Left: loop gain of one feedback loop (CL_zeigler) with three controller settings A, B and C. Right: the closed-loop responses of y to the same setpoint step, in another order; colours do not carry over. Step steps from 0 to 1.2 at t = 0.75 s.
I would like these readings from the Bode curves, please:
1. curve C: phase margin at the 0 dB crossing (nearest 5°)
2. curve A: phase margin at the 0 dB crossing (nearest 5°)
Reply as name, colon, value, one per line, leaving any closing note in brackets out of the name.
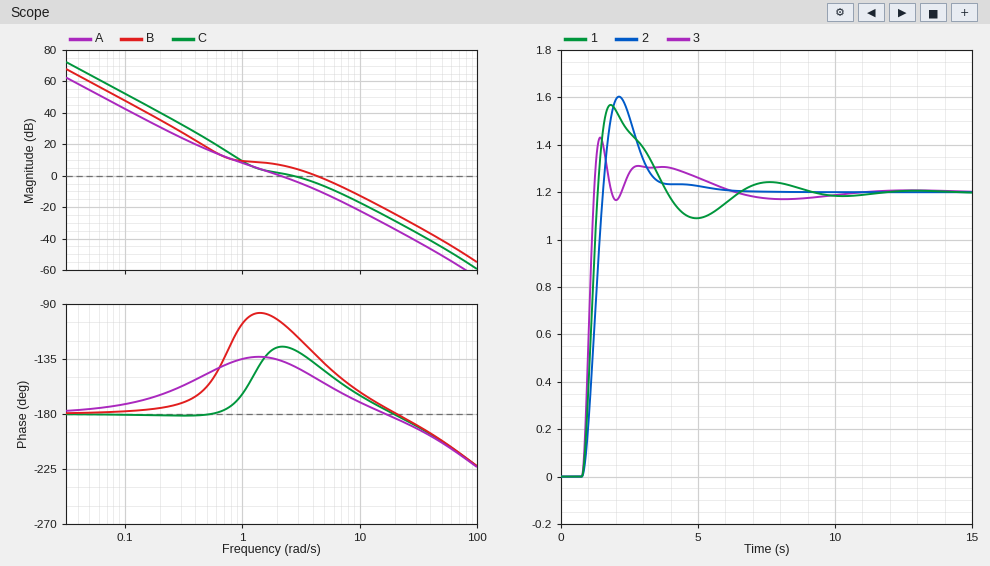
curve C: phase margin at the 0 dB crossing: 55°
curve A: phase margin at the 0 dB crossing: 45°
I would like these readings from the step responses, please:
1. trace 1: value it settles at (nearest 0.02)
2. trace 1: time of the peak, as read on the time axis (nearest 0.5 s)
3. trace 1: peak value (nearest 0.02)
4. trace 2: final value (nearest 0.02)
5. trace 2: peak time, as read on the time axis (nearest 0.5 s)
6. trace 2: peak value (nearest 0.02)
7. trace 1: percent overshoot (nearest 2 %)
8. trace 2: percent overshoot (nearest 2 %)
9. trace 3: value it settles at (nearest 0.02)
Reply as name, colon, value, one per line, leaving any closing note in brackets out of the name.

trace 1: value it settles at: 1.20
trace 1: time of the peak, as read on the time axis: 2.0 s
trace 1: peak value: 1.56
trace 2: final value: 1.20
trace 2: peak time, as read on the time axis: 2.0 s
trace 2: peak value: 1.60
trace 1: percent overshoot: 30 %
trace 2: percent overshoot: 34 %
trace 3: value it settles at: 1.20
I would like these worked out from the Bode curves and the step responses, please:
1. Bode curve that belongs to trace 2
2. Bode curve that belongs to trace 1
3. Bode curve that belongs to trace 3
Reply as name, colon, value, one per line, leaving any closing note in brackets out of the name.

Bode curve that belongs to trace 2: A
Bode curve that belongs to trace 1: C
Bode curve that belongs to trace 3: B
